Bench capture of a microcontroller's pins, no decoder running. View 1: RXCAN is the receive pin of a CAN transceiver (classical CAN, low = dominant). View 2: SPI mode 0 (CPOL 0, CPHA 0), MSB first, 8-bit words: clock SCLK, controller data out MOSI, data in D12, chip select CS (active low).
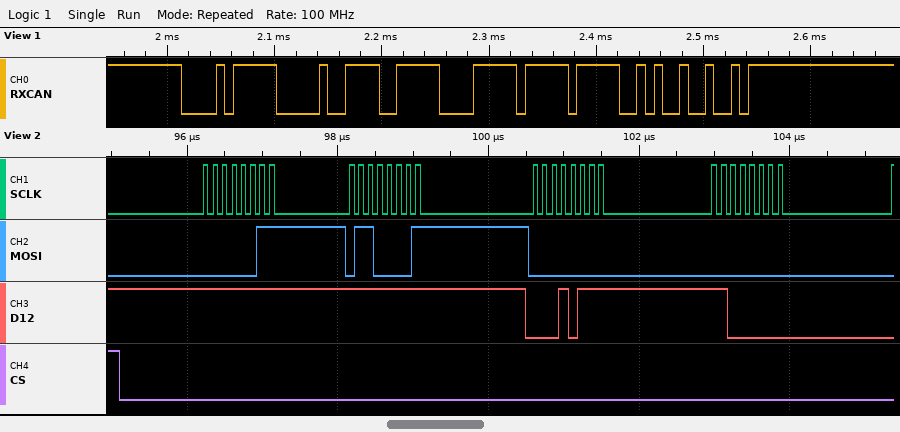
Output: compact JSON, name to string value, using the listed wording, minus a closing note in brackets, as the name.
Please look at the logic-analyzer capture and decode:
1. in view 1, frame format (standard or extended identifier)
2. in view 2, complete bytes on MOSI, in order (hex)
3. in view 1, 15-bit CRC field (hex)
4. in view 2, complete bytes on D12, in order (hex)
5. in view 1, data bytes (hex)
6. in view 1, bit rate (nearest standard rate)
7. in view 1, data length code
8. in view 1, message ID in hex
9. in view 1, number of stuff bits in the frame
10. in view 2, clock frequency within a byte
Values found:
{"in view 1, frame format": "standard", "in view 2, complete bytes on MOSI, in order": "0x03 0x61 0x00 0x00", "in view 1, 15-bit CRC field": "0x7524", "in view 2, complete bytes on D12, in order": "0xFF 0xFF 0x17 0xC0", "in view 1, data bytes": "CF 8F FF", "in view 1, bit rate": "125 kbit/s", "in view 1, data length code": "3", "in view 1, message ID in hex": "0x0BE", "in view 1, number of stuff bits in the frame": "6", "in view 2, clock frequency within a byte": "8 MHz"}
